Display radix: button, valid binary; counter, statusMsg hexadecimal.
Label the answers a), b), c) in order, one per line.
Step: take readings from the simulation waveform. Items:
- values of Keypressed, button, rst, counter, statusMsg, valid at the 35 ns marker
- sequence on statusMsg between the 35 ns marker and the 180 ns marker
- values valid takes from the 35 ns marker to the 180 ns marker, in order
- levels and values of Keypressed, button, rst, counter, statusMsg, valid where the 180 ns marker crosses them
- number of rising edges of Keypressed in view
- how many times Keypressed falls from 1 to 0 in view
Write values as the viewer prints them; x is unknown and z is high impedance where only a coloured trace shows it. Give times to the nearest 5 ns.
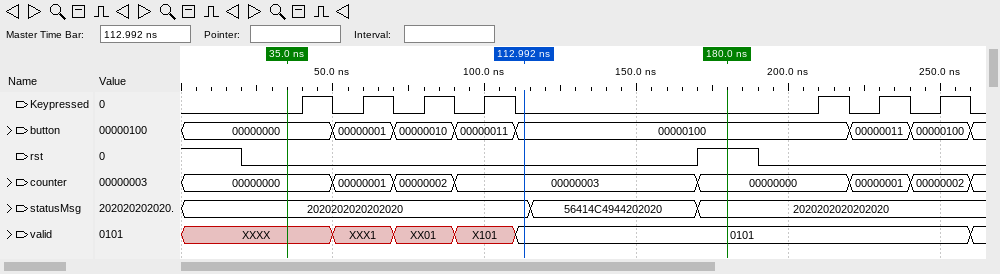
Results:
a) Keypressed=0, button=00000000, rst=0, counter=00000000, statusMsg=2020202020202020, valid=XXXX
b) 2020202020202020, 56414C4944202020, 2020202020202020
c) XXXX, XXX1, XX01, X101, 0101
d) Keypressed=0, button=00000100, rst=1, counter=00000000, statusMsg=2020202020202020, valid=0101
e) 7
f) 7
